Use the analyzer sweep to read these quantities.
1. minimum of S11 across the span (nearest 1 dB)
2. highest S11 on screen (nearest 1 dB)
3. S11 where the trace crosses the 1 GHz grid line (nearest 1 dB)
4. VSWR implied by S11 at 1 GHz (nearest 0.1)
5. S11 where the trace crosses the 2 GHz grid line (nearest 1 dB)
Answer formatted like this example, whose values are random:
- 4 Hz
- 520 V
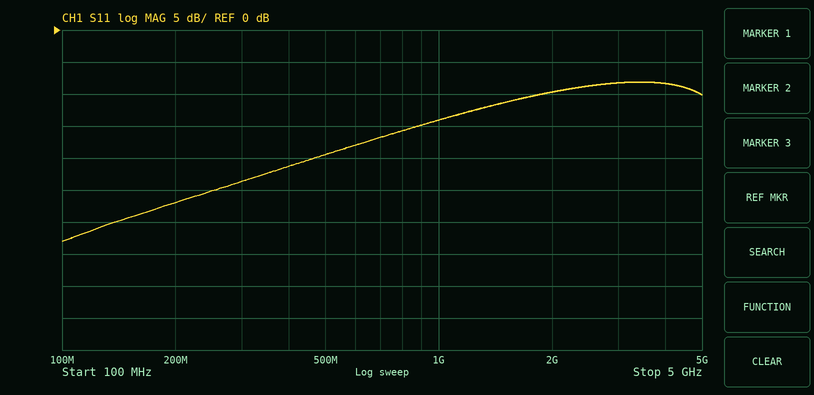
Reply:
- -33 dB
- -8 dB
- -14 dB
- 1.5
- -10 dB
